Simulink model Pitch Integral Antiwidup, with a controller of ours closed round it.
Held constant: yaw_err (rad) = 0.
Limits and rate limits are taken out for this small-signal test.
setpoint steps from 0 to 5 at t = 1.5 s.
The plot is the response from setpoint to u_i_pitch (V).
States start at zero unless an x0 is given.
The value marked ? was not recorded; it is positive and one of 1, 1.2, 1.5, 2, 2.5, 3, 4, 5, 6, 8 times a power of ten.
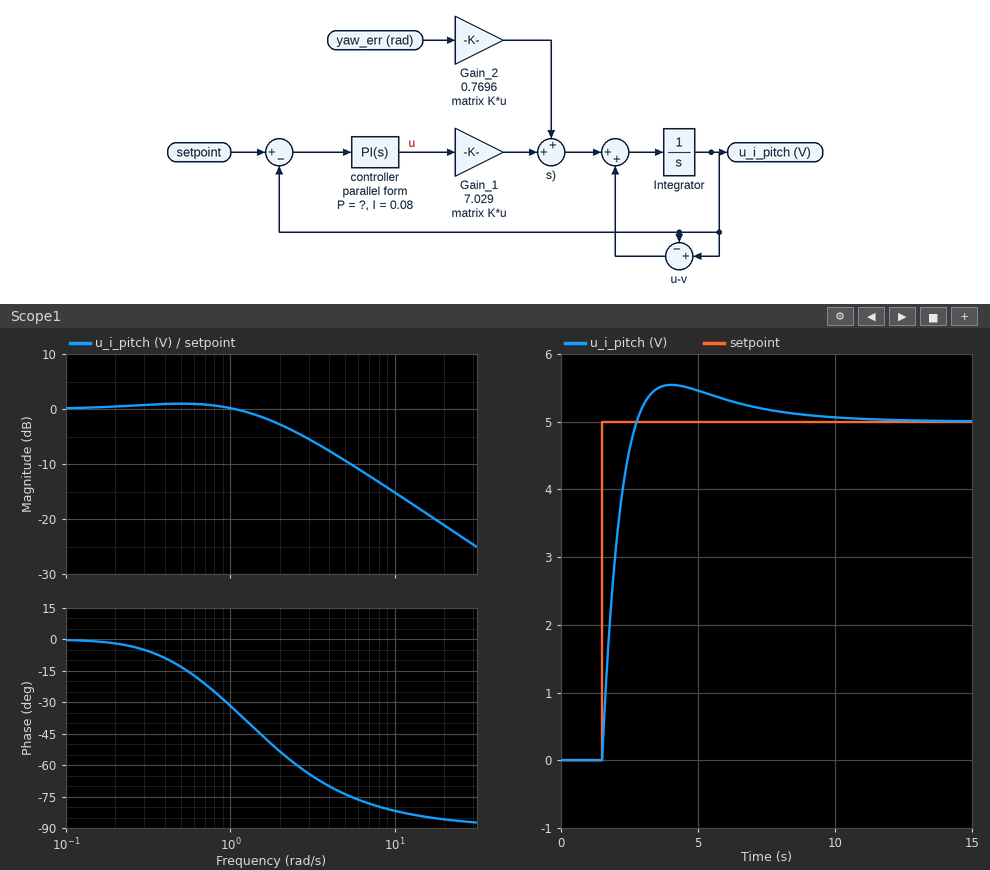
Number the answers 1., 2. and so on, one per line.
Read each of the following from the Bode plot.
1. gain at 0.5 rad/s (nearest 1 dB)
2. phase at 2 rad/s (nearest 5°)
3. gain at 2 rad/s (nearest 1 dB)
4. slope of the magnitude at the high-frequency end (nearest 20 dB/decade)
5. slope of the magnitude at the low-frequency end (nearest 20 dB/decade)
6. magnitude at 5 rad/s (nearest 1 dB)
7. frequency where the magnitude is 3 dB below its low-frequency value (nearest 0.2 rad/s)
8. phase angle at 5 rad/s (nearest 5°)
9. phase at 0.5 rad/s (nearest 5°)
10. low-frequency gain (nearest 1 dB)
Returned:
1. 1 dB
2. -55°
3. -3 dB
4. -20 dB/decade
5. 0 dB/decade
6. -9 dB
7. 2.0 rad/s
8. -75°
9. -15°
10. 0 dB
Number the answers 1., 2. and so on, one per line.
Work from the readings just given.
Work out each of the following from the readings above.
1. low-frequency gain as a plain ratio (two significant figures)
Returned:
1. 1.0
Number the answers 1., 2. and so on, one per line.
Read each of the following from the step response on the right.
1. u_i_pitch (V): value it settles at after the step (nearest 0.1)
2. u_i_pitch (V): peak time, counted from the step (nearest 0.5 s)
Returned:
1. 5.0
2. 2.5 s
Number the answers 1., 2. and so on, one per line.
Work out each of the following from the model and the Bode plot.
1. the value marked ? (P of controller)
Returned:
1. 0.25
